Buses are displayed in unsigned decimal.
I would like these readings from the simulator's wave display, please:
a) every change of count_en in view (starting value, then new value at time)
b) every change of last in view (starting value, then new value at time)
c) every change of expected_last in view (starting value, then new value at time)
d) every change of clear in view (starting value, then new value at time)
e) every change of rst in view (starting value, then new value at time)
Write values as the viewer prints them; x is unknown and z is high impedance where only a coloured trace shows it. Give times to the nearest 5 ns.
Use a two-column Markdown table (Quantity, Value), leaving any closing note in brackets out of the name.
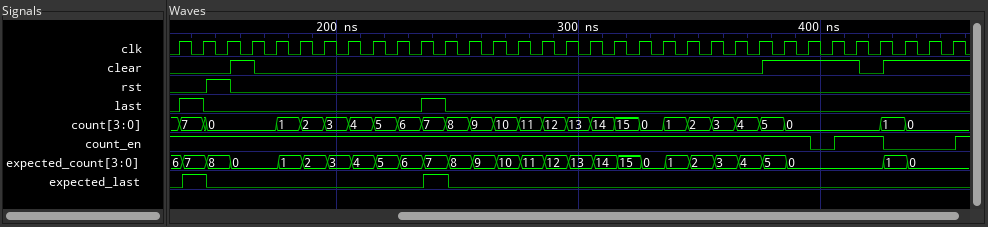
| Quantity | Value |
|---|---|
| every change of count_en in view | 1, 0 at 395 ns, 1 at 405 ns, 0 at 425 ns, 1 at 455 ns |
| every change of last in view | 0, 1 at 135 ns, 0 at 145 ns, 1 at 235 ns, 0 at 245 ns |
| every change of expected_last in view | 0, 1 at 135 ns, 0 at 145 ns, 1 at 235 ns, 0 at 245 ns |
| every change of clear in view | 0, 1 at 155 ns, 0 at 165 ns, 1 at 375 ns, 0 at 415 ns, 1 at 425 ns |
| every change of rst in view | 0, 1 at 145 ns, 0 at 155 ns |
